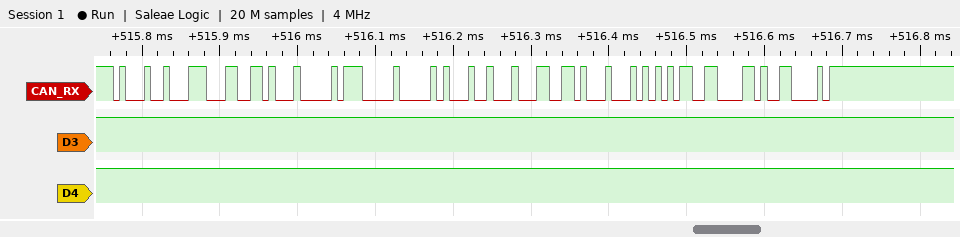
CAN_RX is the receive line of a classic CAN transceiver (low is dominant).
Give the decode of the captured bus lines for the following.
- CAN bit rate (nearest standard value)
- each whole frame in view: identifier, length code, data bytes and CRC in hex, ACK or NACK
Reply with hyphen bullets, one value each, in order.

- 125 kbit/s
- ID 11223344, DLC 7, data 00 11 22 33 44 55 66, CRC 0D30, ACK
